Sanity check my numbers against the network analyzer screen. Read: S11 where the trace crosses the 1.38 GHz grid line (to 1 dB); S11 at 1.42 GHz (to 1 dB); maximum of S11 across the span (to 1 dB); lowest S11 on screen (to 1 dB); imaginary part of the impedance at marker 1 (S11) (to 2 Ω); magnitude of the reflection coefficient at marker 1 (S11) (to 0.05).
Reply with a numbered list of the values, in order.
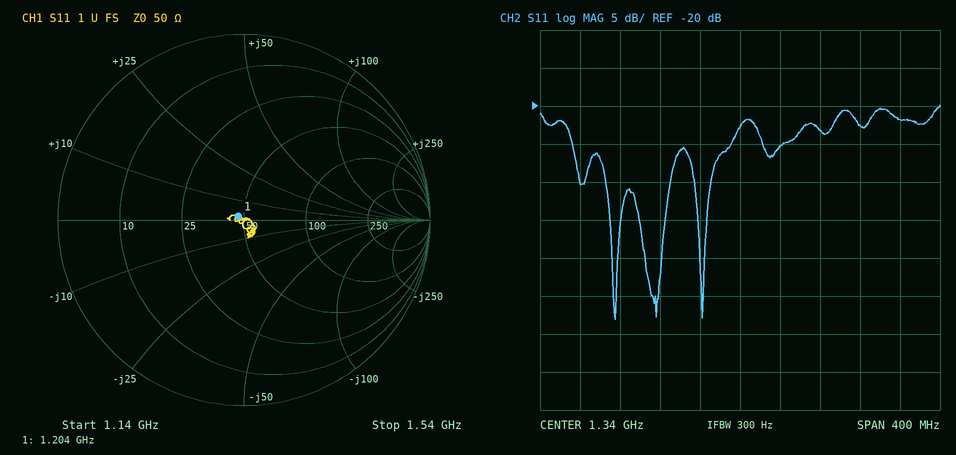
1. -25 dB
2. -23 dB
3. -20 dB
4. -48 dB
5. +2 Ω
6. 0.05
